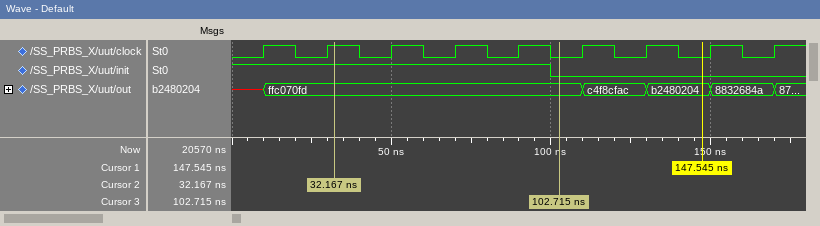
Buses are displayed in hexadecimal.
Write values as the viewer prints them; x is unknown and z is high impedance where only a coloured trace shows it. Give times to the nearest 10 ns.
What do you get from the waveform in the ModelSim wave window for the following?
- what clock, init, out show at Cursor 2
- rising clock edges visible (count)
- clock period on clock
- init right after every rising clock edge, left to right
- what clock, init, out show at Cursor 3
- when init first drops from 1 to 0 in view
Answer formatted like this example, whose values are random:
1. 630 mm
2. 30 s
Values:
1. clock=1, init=1, out=ffc070fd
2. 9
3. 20 ns
4. 1 1 1 1 1 0 0 0 0
5. clock=0, init=0, out=ffc070fd
6. 100 ns
